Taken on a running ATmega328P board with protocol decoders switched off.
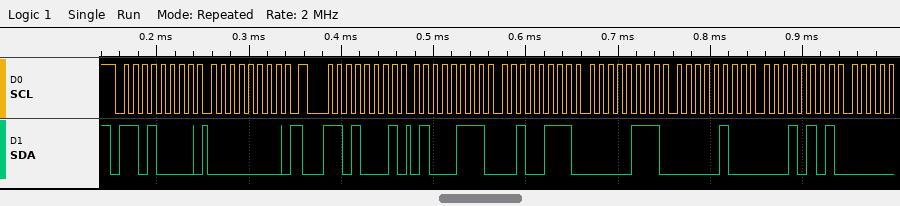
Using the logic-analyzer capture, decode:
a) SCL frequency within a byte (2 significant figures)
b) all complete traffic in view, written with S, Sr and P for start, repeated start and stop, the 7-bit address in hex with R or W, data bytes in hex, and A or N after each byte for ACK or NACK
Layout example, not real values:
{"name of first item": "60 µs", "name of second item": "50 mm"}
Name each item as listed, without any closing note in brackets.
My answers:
{"SCL frequency within a byte": "100 kHz", "all complete traffic in view, written with S, Sr and P for start, repeated start and stop, the 7-bit address in hex with R or W, data bytes in hex, and A or N after each byte for ACK or NACK": "S 68W A 00 A Sr 68R A 47 A 27 A 07 A 04 A 15 A"}
